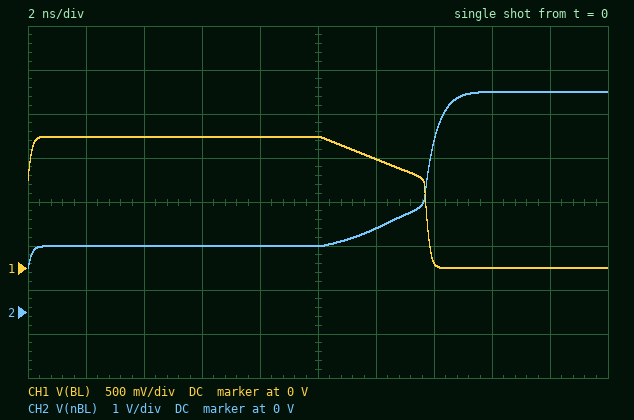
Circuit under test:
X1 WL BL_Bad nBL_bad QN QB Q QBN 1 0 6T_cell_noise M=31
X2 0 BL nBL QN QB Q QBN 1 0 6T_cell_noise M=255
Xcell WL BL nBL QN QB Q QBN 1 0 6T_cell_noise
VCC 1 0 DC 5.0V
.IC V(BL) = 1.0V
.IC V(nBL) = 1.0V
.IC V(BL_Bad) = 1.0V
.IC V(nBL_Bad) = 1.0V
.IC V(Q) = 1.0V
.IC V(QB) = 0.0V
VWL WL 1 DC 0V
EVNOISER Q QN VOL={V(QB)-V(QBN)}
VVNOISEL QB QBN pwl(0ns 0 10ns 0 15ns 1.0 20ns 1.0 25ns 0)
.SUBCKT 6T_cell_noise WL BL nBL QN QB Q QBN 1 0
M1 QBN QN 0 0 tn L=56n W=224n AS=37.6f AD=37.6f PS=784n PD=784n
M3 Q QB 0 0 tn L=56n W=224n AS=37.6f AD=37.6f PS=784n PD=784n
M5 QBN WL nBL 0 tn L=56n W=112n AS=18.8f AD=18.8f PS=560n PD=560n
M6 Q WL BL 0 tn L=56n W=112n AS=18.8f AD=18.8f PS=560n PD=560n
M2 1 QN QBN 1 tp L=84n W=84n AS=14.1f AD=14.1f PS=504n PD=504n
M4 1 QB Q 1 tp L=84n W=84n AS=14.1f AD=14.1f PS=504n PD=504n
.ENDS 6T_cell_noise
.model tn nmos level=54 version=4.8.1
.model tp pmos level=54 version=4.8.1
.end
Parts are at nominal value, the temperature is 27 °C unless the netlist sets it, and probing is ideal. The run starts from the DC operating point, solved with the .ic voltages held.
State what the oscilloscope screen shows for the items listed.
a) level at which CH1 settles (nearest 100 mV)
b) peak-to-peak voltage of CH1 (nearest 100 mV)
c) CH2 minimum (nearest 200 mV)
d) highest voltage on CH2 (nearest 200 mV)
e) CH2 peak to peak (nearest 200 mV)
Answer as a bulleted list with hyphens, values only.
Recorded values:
- 0 V
- 1.5 V
- 1.0 V
- 5.0 V
- 4.0 V
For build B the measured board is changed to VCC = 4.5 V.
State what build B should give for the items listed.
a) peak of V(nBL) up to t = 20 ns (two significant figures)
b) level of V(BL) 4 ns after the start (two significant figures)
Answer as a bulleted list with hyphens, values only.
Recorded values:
- 4.5 V
- 1.2 V
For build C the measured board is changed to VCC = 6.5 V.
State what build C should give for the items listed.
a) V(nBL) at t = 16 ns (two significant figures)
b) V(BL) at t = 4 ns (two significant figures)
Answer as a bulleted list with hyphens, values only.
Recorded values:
- 2.5 V
- 2.4 V
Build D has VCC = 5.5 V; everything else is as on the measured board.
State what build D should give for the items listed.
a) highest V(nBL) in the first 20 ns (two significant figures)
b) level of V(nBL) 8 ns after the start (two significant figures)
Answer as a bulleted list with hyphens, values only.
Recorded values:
- 2.4 V
- 1.8 V
